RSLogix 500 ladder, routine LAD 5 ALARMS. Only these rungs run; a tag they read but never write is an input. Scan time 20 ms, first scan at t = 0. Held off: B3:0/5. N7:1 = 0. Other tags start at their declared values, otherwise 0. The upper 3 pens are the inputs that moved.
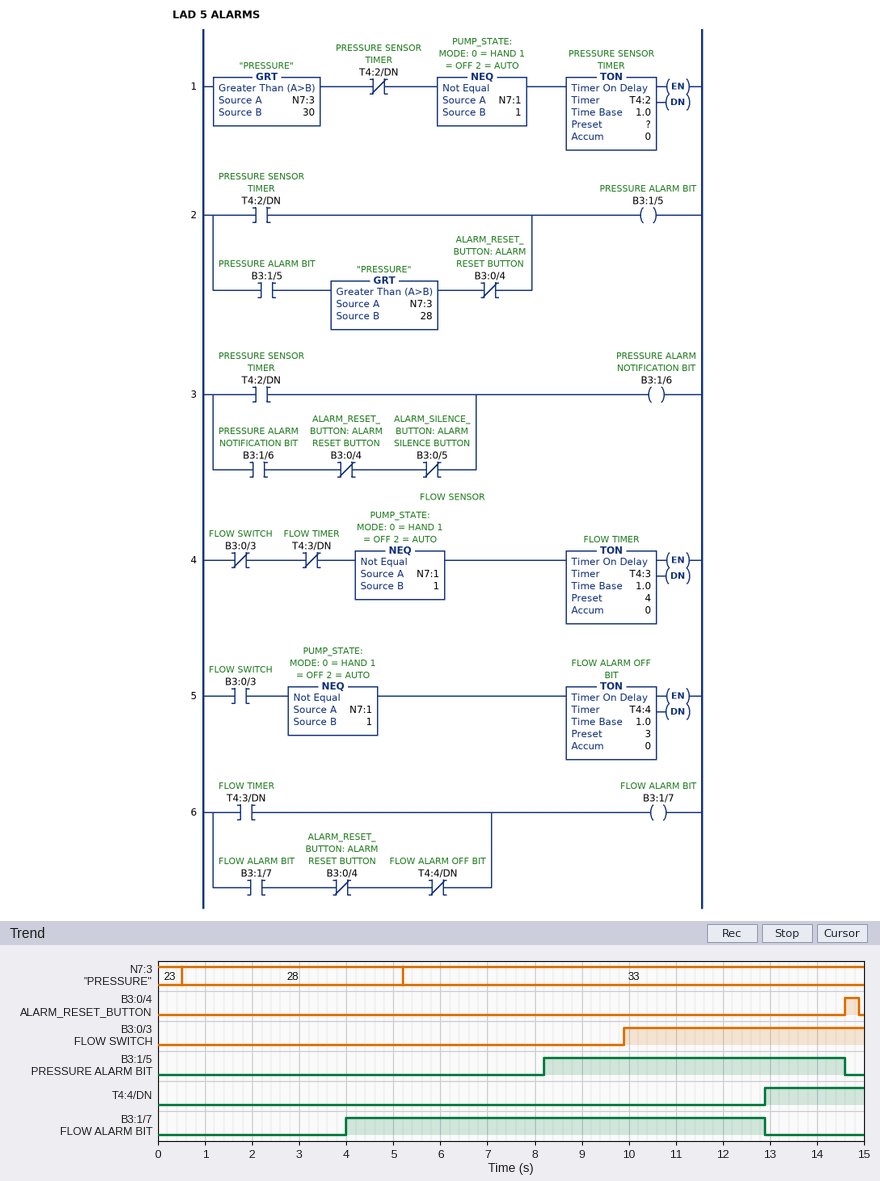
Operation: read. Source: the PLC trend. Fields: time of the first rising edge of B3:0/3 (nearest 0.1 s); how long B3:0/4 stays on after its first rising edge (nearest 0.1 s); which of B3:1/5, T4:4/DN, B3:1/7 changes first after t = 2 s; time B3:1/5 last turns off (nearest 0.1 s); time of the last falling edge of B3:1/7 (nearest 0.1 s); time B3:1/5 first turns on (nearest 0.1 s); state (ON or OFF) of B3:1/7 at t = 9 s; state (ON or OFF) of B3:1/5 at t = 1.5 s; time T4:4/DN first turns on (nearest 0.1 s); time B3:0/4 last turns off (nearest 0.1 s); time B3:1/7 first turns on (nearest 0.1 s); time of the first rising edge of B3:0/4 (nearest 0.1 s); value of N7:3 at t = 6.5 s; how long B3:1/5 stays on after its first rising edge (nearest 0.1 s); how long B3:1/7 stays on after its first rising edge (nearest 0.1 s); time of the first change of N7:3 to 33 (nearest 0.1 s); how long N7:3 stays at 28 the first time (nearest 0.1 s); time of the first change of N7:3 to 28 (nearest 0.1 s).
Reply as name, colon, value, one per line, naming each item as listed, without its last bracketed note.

time of the first rising edge of B3:0/3: 9.9 s
how long B3:0/4 stays on after its first rising edge: 0.3 s
which of B3:1/5, T4:4/DN, B3:1/7 changes first after t = 2 s: B3:1/7
time B3:1/5 last turns off: 14.6 s
time of the last falling edge of B3:1/7: 12.9 s
time B3:1/5 first turns on: 8.2 s
state (ON or OFF) of B3:1/7 at t = 9 s: ON
state (ON or OFF) of B3:1/5 at t = 1.5 s: OFF
time T4:4/DN first turns on: 12.9 s
time B3:0/4 last turns off: 14.9 s
time B3:1/7 first turns on: 4.0 s
time of the first rising edge of B3:0/4: 14.6 s
value of N7:3 at t = 6.5 s: 33
how long B3:1/5 stays on after its first rising edge: 6.4 s
how long B3:1/7 stays on after its first rising edge: 8.9 s
time of the first change of N7:3 to 33: 5.2 s
how long N7:3 stays at 28 the first time: 4.7 s
time of the first change of N7:3 to 28: 0.5 s
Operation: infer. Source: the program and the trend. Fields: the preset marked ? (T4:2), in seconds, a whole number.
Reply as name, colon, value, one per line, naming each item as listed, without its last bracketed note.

the preset marked ? (T4:2), in seconds, a whole number: 3 s
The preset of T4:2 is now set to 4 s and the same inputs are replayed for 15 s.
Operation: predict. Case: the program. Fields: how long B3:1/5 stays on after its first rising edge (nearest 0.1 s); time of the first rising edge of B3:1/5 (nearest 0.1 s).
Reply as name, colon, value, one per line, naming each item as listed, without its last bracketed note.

how long B3:1/5 stays on after its first rising edge: 5.4 s
time of the first rising edge of B3:1/5: 9.2 s
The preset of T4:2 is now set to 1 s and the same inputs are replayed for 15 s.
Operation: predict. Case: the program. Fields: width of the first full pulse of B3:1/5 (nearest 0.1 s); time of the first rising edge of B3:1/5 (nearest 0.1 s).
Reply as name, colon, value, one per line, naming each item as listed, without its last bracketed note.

width of the first full pulse of B3:1/5: 8.4 s
time of the first rising edge of B3:1/5: 6.2 s
